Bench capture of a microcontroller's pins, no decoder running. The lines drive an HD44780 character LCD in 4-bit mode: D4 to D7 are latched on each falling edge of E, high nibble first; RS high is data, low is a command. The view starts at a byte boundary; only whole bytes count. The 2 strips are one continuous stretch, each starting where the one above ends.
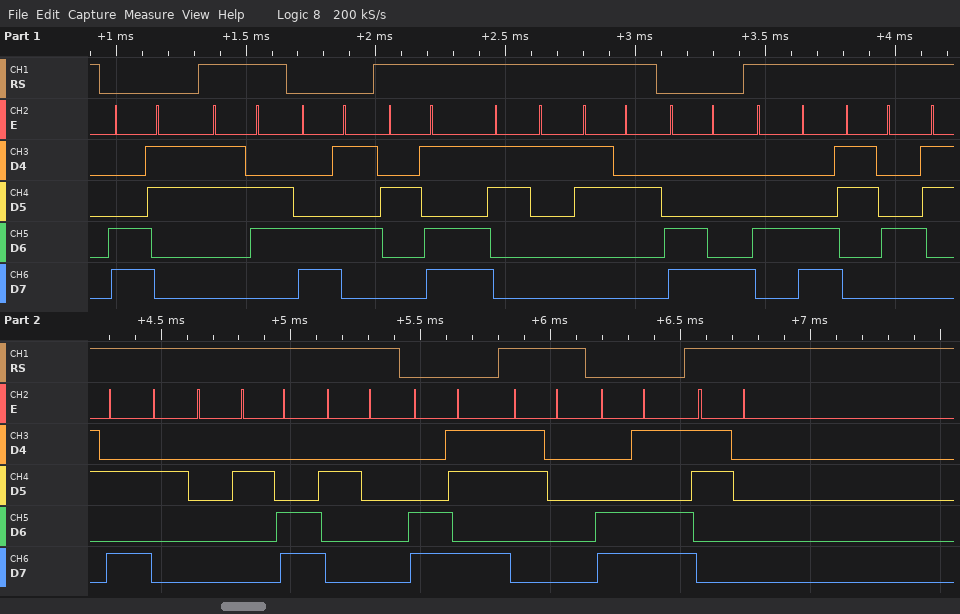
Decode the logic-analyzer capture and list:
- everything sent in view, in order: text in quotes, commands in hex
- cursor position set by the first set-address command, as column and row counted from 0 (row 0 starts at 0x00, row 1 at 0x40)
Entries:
0xC3 "6" 0xC5 "-12" 0xC8 "L4: , " 0xCB "0" 0xCD "0"
column 3, row 1
